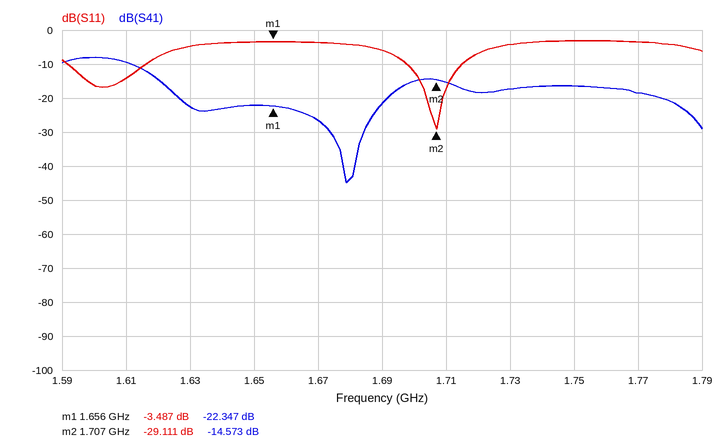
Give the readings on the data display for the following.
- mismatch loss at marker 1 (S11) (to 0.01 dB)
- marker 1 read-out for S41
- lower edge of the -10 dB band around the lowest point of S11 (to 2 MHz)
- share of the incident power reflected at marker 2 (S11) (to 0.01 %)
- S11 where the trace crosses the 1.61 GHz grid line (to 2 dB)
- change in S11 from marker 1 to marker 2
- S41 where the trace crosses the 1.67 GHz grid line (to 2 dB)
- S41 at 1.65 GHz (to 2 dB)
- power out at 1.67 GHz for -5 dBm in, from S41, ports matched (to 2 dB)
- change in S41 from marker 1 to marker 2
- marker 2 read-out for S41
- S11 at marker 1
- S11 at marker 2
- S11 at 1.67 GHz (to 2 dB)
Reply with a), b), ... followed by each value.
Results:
a) 2.58 dB
b) -22.347 dB
c) 1.698 GHz
d) 0.12 %
e) -14 dB
f) -25.624 dB
g) -26 dB
h) -22 dB
i) -32 dBm
j) 7.774 dB
k) -14.573 dB
l) -3.487 dB
m) -29.111 dB
n) -4 dB
